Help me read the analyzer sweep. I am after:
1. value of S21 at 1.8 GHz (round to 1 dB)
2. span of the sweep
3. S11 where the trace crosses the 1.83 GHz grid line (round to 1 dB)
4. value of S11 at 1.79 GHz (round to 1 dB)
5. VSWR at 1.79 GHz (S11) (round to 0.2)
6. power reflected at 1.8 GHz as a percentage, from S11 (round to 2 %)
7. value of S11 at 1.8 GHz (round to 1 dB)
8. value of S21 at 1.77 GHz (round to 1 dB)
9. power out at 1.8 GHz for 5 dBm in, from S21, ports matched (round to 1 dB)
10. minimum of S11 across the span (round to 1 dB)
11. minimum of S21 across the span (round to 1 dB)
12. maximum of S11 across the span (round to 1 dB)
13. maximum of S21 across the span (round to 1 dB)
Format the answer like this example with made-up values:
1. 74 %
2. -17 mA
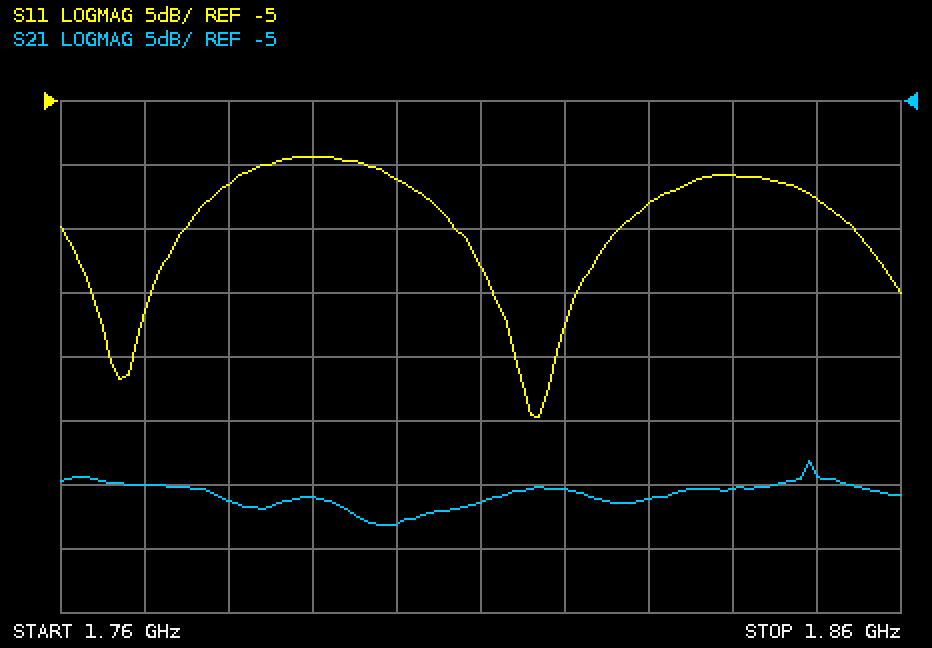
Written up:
1. -38 dB
2. 100 MHz
3. -13 dB
4. -9 dB
5. 2.0
6. 8 %
7. -11 dB
8. -35 dB
9. -33 dBm
10. -30 dB
11. -38 dB
12. -9 dB
13. -33 dB
